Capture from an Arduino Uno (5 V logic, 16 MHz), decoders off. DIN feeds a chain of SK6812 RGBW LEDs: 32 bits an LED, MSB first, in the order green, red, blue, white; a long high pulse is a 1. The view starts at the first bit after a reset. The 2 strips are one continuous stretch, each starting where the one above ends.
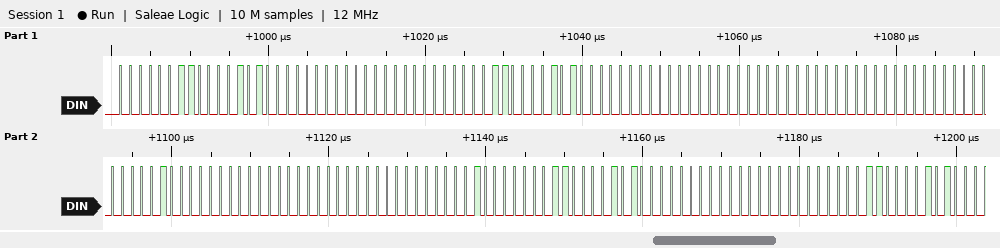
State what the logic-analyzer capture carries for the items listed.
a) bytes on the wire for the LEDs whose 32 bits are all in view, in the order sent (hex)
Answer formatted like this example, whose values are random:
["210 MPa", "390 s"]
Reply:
["03 0A 00 00 03 0A 00 00 00 00 00 02 00 00 00 02 03 0A 00 00"]
